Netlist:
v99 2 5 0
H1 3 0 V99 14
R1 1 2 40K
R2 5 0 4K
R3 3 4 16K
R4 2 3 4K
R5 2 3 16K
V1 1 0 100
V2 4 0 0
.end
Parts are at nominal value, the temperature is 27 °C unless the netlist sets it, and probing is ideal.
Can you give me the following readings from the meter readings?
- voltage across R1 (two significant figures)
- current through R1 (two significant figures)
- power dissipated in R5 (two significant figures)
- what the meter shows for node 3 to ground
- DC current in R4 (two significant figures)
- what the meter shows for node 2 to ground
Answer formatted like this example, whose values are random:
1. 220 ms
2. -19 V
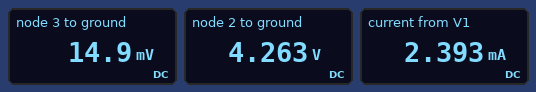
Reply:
1. 96 V
2. 2.4 mA
3. 1.1 mW
4. 14.9 mV
5. 1.1 mA
6. 4.263 V
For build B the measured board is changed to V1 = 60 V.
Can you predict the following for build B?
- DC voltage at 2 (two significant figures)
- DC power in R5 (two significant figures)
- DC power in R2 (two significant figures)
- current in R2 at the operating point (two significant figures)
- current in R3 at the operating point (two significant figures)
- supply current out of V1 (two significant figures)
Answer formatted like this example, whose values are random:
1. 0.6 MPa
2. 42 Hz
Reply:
1. 2.6 V
2. 410 µW
3. 1.6 mW
4. 640 µA
5. 560 nA
6. 1.4 mA
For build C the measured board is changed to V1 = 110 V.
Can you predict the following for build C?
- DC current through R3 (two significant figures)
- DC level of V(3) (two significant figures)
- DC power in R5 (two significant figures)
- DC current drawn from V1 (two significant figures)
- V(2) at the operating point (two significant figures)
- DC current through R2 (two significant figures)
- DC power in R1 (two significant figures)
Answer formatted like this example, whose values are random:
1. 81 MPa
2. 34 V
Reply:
1. 1.0 µA
2. 16 mV
3. 1.4 mW
4. 2.6 mA
5. 4.7 V
6. 1.2 mA
7. 280 mW
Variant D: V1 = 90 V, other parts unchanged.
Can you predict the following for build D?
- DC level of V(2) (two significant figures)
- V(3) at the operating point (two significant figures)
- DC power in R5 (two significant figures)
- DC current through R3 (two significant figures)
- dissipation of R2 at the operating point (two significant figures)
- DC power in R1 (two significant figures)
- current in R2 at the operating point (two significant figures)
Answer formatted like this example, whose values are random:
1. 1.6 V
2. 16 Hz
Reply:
1. 3.8 V
2. 13 mV
3. 910 µW
4. 840 nA
5. 3.7 mW
6. 190 mW
7. 960 µA
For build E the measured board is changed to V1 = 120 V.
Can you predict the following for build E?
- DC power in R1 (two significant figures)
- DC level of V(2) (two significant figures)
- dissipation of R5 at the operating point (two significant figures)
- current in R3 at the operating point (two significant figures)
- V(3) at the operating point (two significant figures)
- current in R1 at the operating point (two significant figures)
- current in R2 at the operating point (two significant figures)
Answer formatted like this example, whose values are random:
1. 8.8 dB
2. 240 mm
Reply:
1. 330 mW
2. 5.1 V
3. 1.6 mW
4. 1.1 µA
5. 18 mV
6. 2.9 mA
7. 1.3 mA
